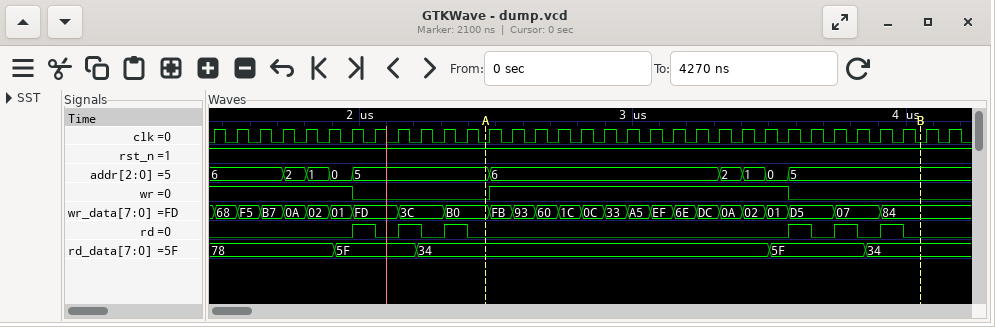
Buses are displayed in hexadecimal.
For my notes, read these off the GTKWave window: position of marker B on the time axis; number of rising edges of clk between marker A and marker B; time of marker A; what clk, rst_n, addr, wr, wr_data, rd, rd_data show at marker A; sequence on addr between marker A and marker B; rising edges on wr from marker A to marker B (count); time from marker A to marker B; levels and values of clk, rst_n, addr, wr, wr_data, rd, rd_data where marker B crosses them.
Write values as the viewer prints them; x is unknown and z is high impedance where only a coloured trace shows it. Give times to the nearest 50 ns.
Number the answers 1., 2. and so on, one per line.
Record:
1. 4050 ns
2. 19
3. 2450 ns
4. clk=0, rst_n=1, addr=5, wr=0, wr_data=B0, rd=0, rd_data=34
5. 5, 6, 2, 1, 0, 5
6. 1
7. 1600 ns
8. clk=0, rst_n=1, addr=5, wr=0, wr_data=84, rd=0, rd_data=34
